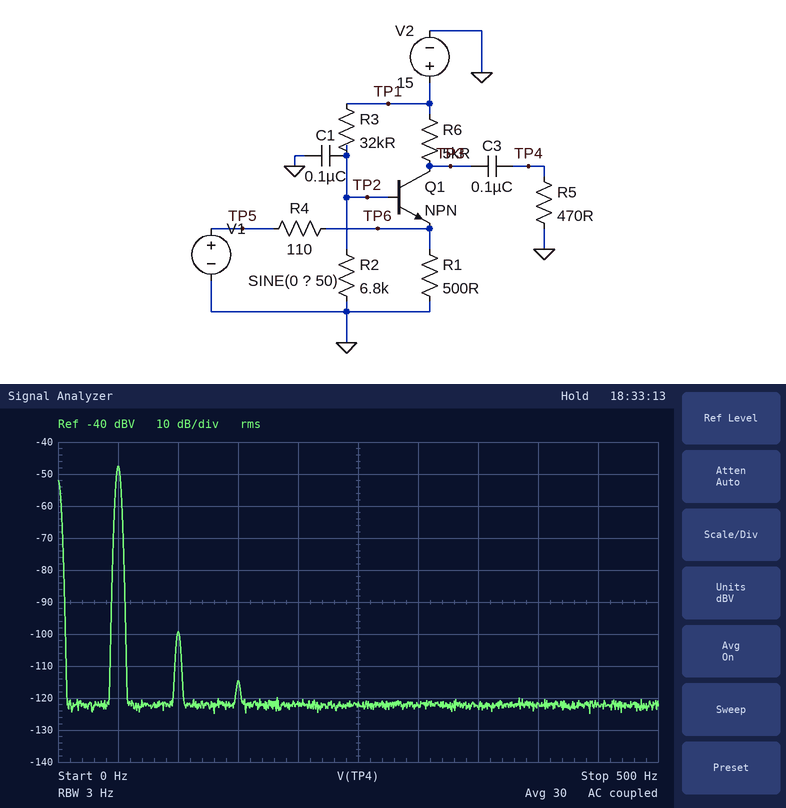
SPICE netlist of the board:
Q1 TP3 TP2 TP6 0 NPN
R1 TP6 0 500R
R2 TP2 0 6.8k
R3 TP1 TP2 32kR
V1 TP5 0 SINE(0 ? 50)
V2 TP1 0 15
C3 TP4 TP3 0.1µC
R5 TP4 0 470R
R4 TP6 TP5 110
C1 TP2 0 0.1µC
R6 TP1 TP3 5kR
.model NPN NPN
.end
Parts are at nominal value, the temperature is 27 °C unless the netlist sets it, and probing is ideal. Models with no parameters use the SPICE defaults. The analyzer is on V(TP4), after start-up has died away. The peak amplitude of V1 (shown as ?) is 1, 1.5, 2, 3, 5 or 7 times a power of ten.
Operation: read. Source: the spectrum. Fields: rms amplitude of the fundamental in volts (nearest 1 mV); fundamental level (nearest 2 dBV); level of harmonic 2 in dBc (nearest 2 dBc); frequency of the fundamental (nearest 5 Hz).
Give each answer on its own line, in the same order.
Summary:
4 mV
-48 dBV
-52 dBc
50 Hz
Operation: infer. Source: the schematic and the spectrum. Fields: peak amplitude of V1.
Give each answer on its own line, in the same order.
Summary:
500 mV
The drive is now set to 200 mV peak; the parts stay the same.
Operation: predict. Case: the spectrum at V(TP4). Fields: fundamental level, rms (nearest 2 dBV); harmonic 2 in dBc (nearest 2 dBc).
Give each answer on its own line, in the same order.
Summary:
-56 dBV
-60 dBc
